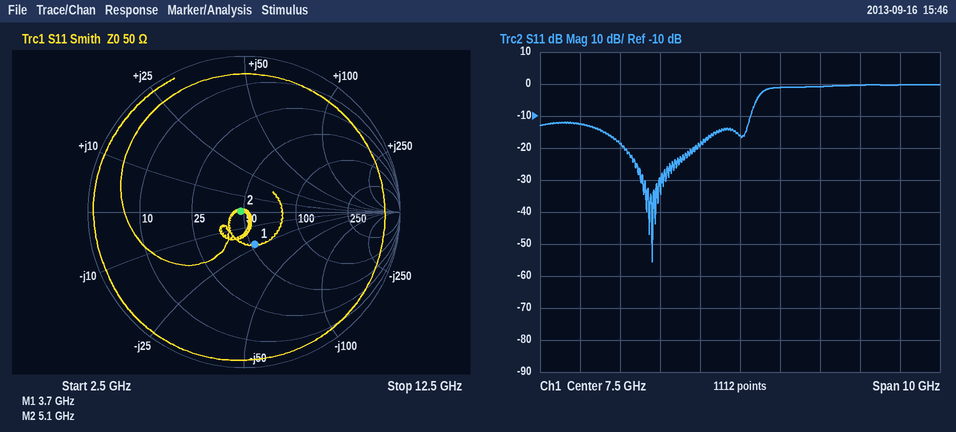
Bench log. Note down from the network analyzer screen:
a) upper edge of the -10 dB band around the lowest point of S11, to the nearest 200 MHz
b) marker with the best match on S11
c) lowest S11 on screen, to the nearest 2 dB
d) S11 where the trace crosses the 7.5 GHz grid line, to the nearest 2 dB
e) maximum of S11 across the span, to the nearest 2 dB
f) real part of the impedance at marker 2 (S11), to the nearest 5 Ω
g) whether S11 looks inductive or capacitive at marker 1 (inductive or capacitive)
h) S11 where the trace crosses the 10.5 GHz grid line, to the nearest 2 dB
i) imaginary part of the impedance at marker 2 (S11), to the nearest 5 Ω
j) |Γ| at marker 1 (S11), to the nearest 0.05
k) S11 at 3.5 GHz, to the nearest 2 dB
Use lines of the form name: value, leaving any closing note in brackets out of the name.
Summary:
upper edge of the -10 dB band around the lowest point of S11, to the nearest 200 MHz: 7.8 GHz
marker with the best match on S11: marker 2
lowest S11 on screen, to the nearest 2 dB: -56 dB
S11 where the trace crosses the 7.5 GHz grid line, to the nearest 2 dB: -16 dB
maximum of S11 across the span, to the nearest 2 dB: 0 dB
real part of the impedance at marker 2 (S11), to the nearest 5 Ω: 50 Ω
whether S11 looks inductive or capacitive at marker 1: capacitive
S11 where the trace crosses the 10.5 GHz grid line, to the nearest 2 dB: 0 dB
imaginary part of the impedance at marker 2 (S11), to the nearest 5 Ω: 0 Ω
|Γ| at marker 1 (S11), to the nearest 0.05: 0.20
S11 at 3.5 GHz, to the nearest 2 dB: -12 dB
